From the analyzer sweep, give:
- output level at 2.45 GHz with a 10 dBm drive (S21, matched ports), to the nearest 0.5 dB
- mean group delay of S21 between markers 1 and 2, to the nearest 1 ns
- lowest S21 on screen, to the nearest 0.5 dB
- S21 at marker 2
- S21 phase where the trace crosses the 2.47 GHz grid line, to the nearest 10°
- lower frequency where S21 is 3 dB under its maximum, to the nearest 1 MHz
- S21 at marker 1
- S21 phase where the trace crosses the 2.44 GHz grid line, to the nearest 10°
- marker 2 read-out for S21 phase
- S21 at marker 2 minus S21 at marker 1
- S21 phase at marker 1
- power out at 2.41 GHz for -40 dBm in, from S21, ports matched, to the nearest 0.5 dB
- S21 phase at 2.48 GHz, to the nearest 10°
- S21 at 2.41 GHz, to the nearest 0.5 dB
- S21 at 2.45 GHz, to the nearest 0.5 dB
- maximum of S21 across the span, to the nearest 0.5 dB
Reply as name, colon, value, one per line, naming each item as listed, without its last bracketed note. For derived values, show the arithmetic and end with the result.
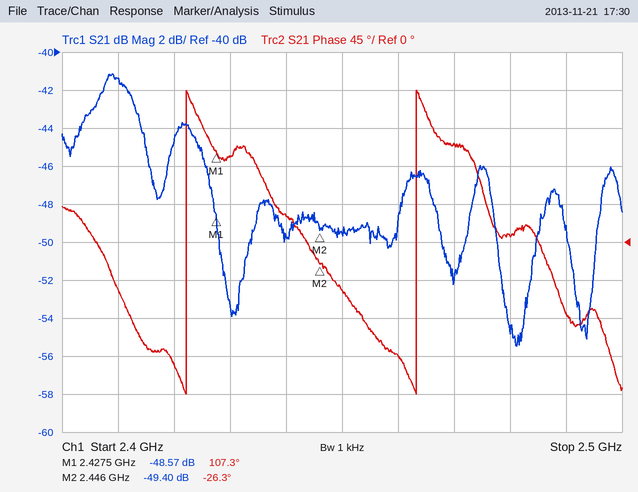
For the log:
output level at 2.45 GHz with a 10 dBm drive (S21, matched ports), to the nearest 0.5 dB: 10 dBm + (-49.5 dB) = -39.5 dBm
mean group delay of S21 between markers 1 and 2, to the nearest 1 ns: −(-26.3° − (107.3°))/(360° × 18.5 MHz) ≈ 20 ns
lowest S21 on screen, to the nearest 0.5 dB: -55.5 dB
S21 at marker 2: -49.40 dB
S21 phase where the trace crosses the 2.47 GHz grid line, to the nearest 10°: 120°
lower frequency where S21 is 3 dB under its maximum, to the nearest 1 MHz: 2.403 GHz
S21 at marker 1: -48.57 dB
S21 phase where the trace crosses the 2.44 GHz grid line, to the nearest 10°: 30°
marker 2 read-out for S21 phase: -26.3°
S21 at marker 2 minus S21 at marker 1: -49.4 − (-48.57) = -0.83 dB
S21 phase at marker 1: 107.3°
power out at 2.41 GHz for -40 dBm in, from S21, ports matched, to the nearest 0.5 dB: -40 dBm + (-41.5 dB) = -81.5 dBm
S21 phase at 2.48 GHz, to the nearest 10°: 10°
S21 at 2.41 GHz, to the nearest 0.5 dB: -41.5 dB
S21 at 2.45 GHz, to the nearest 0.5 dB: -49.5 dB
maximum of S21 across the span, to the nearest 0.5 dB: -41.0 dB
